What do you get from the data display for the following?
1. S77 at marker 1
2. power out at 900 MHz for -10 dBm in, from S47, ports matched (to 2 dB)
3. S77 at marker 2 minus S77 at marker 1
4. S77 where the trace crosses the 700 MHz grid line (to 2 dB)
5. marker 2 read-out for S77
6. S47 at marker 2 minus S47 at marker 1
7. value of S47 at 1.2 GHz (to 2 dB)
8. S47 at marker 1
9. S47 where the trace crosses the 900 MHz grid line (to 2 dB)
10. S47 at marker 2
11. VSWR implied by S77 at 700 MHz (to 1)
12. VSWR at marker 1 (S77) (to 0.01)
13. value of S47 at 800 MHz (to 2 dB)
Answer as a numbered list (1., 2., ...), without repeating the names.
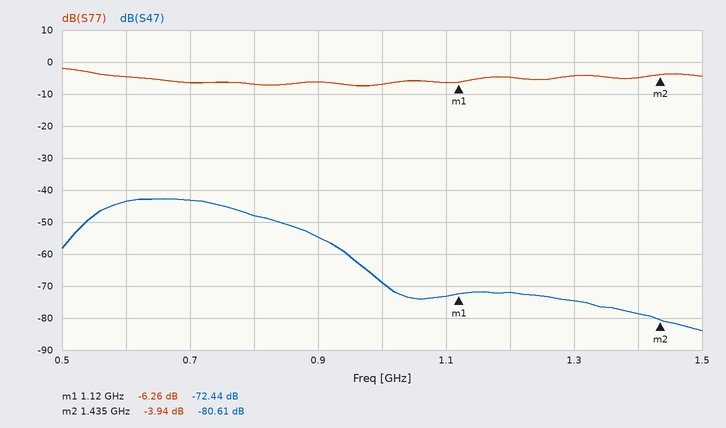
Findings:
1. -6.26 dB
2. -64 dBm
3. 2.32 dB
4. -6 dB
5. -3.94 dB
6. -8.17 dB
7. -72 dB
8. -72.44 dB
9. -54 dB
10. -80.61 dB
11. 3
12. 2.89
13. -48 dB
